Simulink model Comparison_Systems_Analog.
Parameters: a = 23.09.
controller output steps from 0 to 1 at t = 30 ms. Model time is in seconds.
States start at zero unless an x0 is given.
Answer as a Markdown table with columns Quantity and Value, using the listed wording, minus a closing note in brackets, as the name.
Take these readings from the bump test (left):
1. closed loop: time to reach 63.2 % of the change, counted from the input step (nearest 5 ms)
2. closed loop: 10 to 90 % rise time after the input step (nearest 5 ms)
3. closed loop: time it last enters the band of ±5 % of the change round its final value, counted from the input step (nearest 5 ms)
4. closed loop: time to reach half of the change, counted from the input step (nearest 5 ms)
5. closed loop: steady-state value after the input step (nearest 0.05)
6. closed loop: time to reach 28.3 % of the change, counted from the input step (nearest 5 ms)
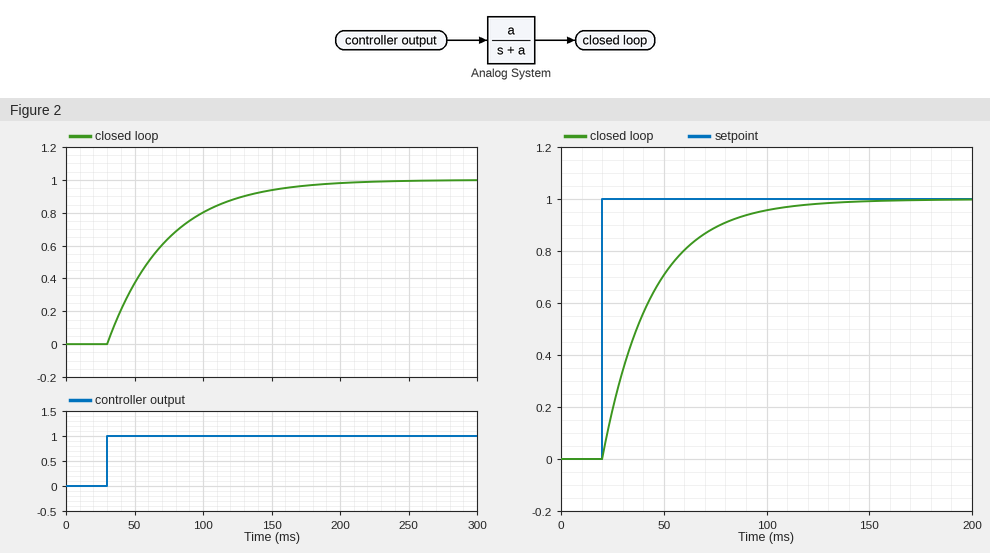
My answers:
| Quantity | Value |
|---|---|
| closed loop: time to reach 63.2 % of the change, counted from the input step | 45 ms |
| closed loop: 10 to 90 % rise time after the input step | 95 ms |
| closed loop: time it last enters the band of ±5 % of the change round its final value, counted from the input step | 130 ms |
| closed loop: time to reach half of the change, counted from the input step | 30 ms |
| closed loop: steady-state value after the input step | 1.00 |
| closed loop: time to reach 28.3 % of the change, counted from the input step | 15 ms |
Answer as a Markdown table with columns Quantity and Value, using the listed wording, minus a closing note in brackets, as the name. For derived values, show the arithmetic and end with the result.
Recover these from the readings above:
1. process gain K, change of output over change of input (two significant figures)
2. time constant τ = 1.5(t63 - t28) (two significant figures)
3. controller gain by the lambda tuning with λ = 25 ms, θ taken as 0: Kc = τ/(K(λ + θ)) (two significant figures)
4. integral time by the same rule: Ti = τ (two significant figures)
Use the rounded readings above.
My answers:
| Quantity | Value |
|---|---|
| process gain K, change of output over change of input | (1 - 0) / 1 = 1.0 |
| time constant τ = 1.5(t63 - t28) | 1.5 × (45 - 15) = 45 ms |
| controller gain by the lambda tuning with λ = 25 ms, θ taken as 0: Kc = τ/(K(λ + θ)) | 45 / (1 × (25 + 0)) = 1.8 |
| integral time by the same rule: Ti = τ | 45 ms |
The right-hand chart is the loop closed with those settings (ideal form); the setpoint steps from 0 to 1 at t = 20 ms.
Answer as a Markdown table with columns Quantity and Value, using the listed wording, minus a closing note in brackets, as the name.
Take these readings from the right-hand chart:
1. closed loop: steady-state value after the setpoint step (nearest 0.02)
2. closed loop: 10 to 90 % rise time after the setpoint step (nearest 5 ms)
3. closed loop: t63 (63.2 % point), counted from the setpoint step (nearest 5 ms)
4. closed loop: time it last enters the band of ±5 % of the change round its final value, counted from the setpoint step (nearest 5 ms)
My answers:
| Quantity | Value |
|---|---|
| closed loop: steady-state value after the setpoint step | 1.00 |
| closed loop: 10 to 90 % rise time after the setpoint step | 55 ms |
| closed loop: t63 (63.2 % point), counted from the setpoint step | 25 ms |
| closed loop: time it last enters the band of ±5 % of the change round its final value, counted from the setpoint step | 75 ms |
